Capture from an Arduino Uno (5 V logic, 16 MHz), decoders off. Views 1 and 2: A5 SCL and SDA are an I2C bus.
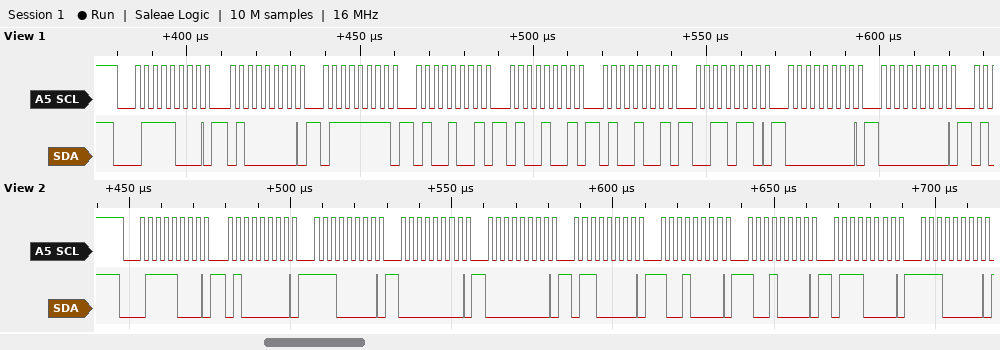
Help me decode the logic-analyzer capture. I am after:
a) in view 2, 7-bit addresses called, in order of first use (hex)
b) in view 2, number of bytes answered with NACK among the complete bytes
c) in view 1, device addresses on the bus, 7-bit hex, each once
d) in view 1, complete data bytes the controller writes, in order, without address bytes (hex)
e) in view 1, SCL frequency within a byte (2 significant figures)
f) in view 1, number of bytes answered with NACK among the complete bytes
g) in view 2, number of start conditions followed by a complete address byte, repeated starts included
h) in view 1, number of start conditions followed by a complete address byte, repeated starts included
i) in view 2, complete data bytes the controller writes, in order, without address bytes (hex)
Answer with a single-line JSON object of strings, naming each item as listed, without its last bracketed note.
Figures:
{"in view 2, 7-bit addresses called, in order of first use": "0x3C", "in view 2, number of bytes answered with NACK among the complete bytes": "0", "in view 1, device addresses on the bus, 7-bit hex, each once": "0x3C", "in view 1, complete data bytes the controller writes, in order, without address bytes": "40 7F 49 49 49 36 00 00", "in view 1, SCL frequency within a byte": "400 kHz", "in view 1, number of bytes answered with NACK among the complete bytes": "0", "in view 2, number of start conditions followed by a complete address byte, repeated starts included": "1", "in view 1, number of start conditions followed by a complete address byte, repeated starts included": "1", "in view 2, complete data bytes the controller writes, in order, without address bytes": "40 E0 00 00 60 90 90 70 E0"}
